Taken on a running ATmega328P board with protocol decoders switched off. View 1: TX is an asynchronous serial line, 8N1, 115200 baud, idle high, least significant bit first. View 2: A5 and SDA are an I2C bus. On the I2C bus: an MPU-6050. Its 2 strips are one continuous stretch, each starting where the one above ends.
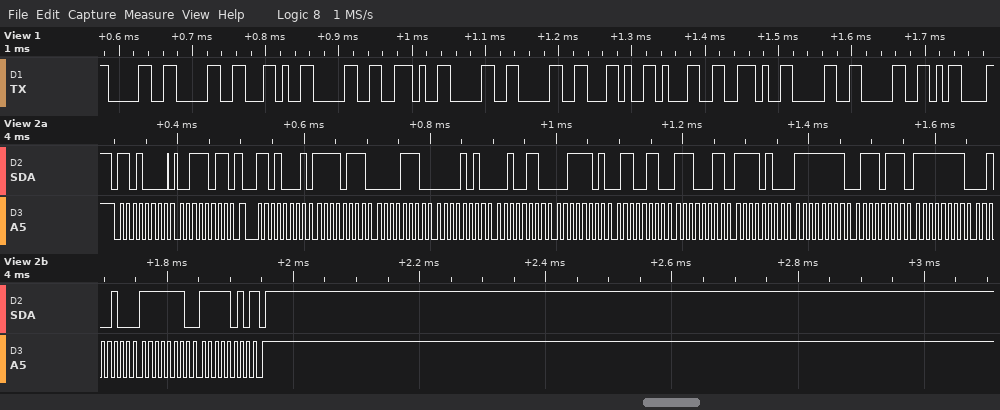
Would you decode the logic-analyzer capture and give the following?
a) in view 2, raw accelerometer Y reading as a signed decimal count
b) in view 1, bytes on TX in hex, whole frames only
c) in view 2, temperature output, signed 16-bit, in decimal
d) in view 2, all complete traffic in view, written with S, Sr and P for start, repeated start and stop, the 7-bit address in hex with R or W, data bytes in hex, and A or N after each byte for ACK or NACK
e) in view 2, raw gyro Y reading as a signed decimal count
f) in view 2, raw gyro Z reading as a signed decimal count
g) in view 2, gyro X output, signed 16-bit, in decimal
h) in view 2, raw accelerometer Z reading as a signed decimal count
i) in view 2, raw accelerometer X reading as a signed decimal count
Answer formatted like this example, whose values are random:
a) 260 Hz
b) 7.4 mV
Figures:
a) 2598
b) 30 30 2C 30 2E 30 30 2C 31 2E 30 30 0D
c) -7180
d) S 68W A 3B A Sr 68R A F7 A 0E A 0A A 26 A 3D A 66 A E3 A F4 A FF A 77 A FF A 24 A FE A FA N P
e) -220
f) -262
g) -137
h) 15718
i) -2290
